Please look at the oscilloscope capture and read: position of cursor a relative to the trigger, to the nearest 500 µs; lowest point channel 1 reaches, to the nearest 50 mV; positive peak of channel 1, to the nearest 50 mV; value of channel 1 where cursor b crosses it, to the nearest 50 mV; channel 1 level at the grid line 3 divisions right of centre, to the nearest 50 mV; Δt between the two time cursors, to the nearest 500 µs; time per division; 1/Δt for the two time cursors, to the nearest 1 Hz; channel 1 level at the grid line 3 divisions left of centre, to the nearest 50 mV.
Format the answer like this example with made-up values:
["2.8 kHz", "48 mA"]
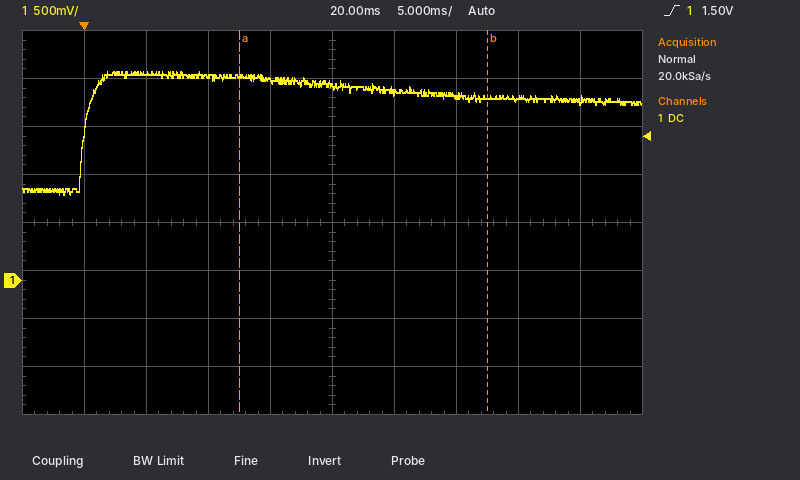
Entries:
["+12.5 ms", "900 mV", "2.15 V", "1.90 V", "1.90 V", "20.0 ms", "5 ms", "50 Hz", "2.15 V"]
